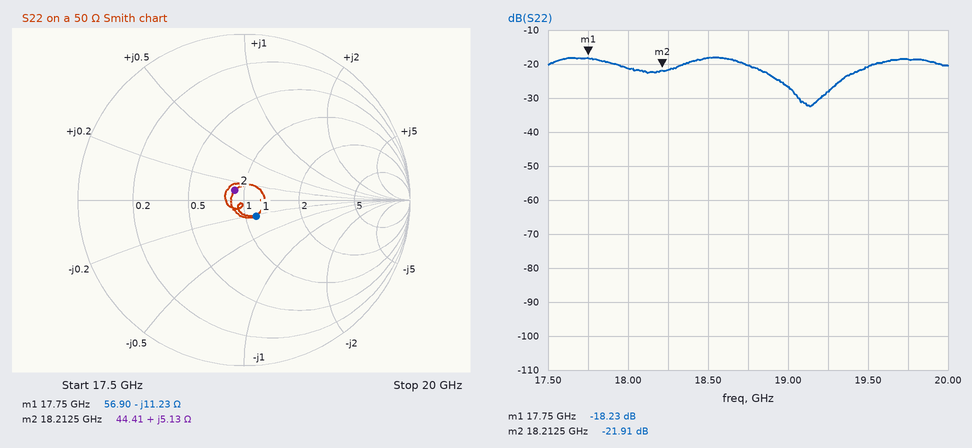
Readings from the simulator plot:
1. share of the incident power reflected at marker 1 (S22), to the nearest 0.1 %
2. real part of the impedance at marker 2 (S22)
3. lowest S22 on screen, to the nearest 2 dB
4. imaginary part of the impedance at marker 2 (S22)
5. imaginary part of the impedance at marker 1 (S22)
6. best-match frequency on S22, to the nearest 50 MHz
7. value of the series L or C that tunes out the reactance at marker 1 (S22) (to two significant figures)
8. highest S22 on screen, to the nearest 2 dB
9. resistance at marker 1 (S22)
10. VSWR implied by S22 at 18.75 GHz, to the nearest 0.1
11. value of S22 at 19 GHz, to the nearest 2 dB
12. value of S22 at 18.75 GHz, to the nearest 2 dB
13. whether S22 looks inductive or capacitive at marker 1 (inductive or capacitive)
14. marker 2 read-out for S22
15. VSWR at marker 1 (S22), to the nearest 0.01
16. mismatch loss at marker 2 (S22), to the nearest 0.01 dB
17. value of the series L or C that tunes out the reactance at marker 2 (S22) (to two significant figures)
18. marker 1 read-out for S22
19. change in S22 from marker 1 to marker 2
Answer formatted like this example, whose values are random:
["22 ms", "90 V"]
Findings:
["1.5 %", "44.41 Ω", "-32 dB", "+5.13 Ω", "-11.23 Ω", "19.15 GHz", "100 pH", "-18 dB", "56.90 Ω", "1.2", "-26 dB", "-20 dB", "capacitive", "-21.91 dB", "1.28", "0.03 dB", "1.7 pF", "-18.23 dB", "-3.68 dB"]
